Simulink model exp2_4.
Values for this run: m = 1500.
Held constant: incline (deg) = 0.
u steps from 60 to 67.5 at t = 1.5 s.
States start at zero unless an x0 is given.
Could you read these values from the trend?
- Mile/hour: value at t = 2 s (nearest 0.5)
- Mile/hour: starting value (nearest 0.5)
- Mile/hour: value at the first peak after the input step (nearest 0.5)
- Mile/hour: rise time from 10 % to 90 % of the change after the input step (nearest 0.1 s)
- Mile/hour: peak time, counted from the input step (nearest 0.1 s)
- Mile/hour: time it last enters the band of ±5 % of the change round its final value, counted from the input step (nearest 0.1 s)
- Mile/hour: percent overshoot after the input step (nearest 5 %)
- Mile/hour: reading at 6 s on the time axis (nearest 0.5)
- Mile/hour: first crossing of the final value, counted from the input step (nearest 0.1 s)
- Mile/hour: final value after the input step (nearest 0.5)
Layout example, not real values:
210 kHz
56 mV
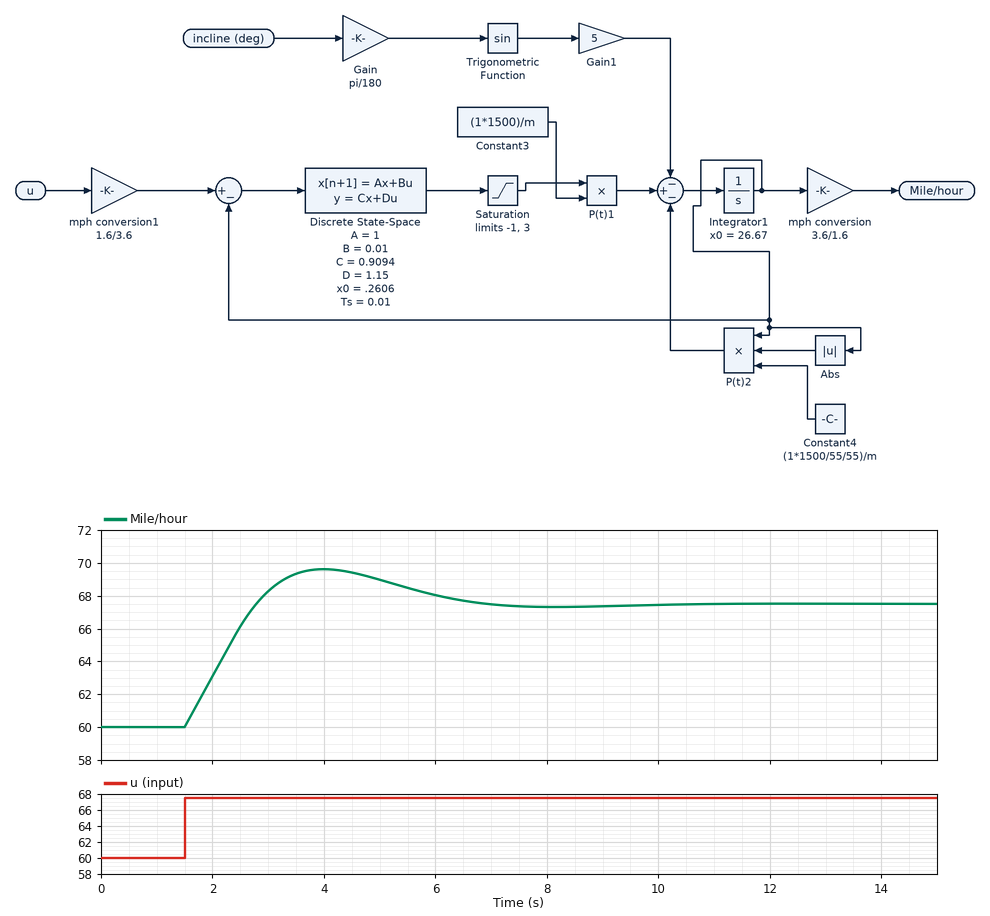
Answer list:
63.0
60.0
69.5
1.0 s
2.5 s
4.7 s
30 %
68.0
1.3 s
67.5
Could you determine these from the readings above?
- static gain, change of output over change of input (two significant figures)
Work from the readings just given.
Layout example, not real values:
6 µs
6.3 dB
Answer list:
1.0
